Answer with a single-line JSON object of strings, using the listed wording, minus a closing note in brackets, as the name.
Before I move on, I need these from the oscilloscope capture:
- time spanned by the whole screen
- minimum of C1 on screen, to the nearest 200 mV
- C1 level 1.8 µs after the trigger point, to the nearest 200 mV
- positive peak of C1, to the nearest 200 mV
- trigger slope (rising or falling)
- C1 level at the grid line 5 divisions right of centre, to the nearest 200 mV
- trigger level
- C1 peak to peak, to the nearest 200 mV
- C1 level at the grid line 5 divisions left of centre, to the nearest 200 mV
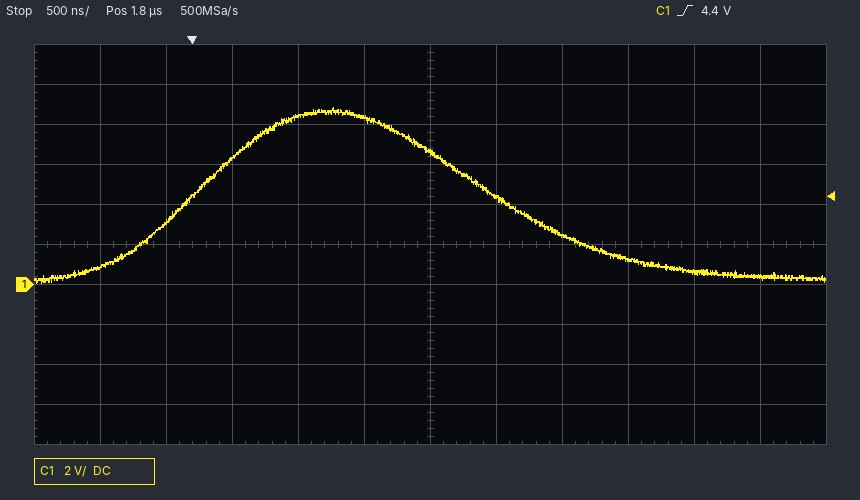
{"time spanned by the whole screen": "6 µs", "minimum of C1 on screen, to the nearest 200 mV": "0.0 V", "C1 level 1.8 µs after the trigger point, to the nearest 200 mV": "6.6 V", "positive peak of C1, to the nearest 200 mV": "8.8 V", "trigger slope": "rising", "C1 level at the grid line 5 divisions right of centre, to the nearest 200 mV": "400 mV", "trigger level": "4.4 V", "C1 peak to peak, to the nearest 200 mV": "8.8 V", "C1 level at the grid line 5 divisions left of centre, to the nearest 200 mV": "800 mV"}
